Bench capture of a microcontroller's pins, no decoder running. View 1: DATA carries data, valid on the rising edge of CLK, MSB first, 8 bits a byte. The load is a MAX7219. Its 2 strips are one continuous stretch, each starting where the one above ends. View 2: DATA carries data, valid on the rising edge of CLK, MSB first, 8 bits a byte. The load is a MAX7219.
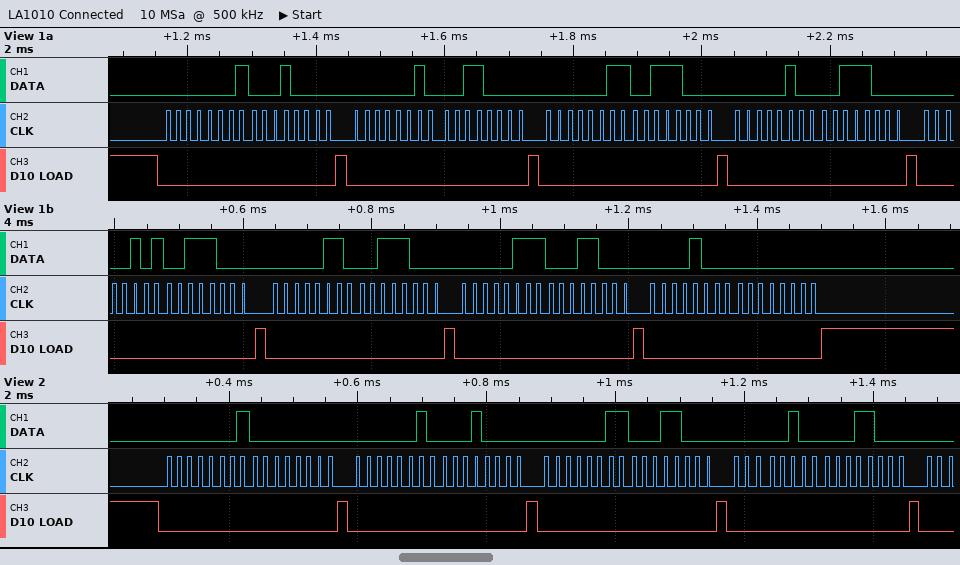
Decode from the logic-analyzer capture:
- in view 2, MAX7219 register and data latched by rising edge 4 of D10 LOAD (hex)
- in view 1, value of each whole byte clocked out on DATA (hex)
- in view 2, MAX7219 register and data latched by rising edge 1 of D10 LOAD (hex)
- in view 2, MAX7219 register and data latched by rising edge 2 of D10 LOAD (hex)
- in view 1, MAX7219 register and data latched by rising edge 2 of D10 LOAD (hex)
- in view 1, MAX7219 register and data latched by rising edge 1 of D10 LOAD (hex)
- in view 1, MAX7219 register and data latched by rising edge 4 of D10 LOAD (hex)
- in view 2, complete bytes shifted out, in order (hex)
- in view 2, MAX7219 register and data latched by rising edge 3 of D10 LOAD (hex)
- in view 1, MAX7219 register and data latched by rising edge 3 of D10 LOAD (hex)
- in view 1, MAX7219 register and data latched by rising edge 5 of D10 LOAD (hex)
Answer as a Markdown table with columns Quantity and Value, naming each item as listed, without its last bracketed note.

| Quantity | Value |
|---|---|
| in view 2, MAX7219 register and data latched by rising edge 4 of D10 LOAD | register 0x4, data 0x18 |
| in view 1, value of each whole byte clocked out on DATA | 01 10 02 30 03 38 04 38 05 38 06 38 07 18 08 00 |
| in view 2, MAX7219 register and data latched by rising edge 1 of D10 LOAD | register 0x1, data 0x00 |
| in view 2, MAX7219 register and data latched by rising edge 2 of D10 LOAD | register 0x2, data 0x10 |
| in view 1, MAX7219 register and data latched by rising edge 2 of D10 LOAD | register 0x2, data 0x30 |
| in view 1, MAX7219 register and data latched by rising edge 1 of D10 LOAD | register 0x1, data 0x10 |
| in view 1, MAX7219 register and data latched by rising edge 4 of D10 LOAD | register 0x4, data 0x38 |
| in view 2, complete bytes shifted out, in order | 01 00 02 10 03 18 04 18 |
| in view 2, MAX7219 register and data latched by rising edge 3 of D10 LOAD | register 0x3, data 0x18 |
| in view 1, MAX7219 register and data latched by rising edge 3 of D10 LOAD | register 0x3, data 0x38 |
| in view 1, MAX7219 register and data latched by rising edge 5 of D10 LOAD | register 0x5, data 0x38 |
